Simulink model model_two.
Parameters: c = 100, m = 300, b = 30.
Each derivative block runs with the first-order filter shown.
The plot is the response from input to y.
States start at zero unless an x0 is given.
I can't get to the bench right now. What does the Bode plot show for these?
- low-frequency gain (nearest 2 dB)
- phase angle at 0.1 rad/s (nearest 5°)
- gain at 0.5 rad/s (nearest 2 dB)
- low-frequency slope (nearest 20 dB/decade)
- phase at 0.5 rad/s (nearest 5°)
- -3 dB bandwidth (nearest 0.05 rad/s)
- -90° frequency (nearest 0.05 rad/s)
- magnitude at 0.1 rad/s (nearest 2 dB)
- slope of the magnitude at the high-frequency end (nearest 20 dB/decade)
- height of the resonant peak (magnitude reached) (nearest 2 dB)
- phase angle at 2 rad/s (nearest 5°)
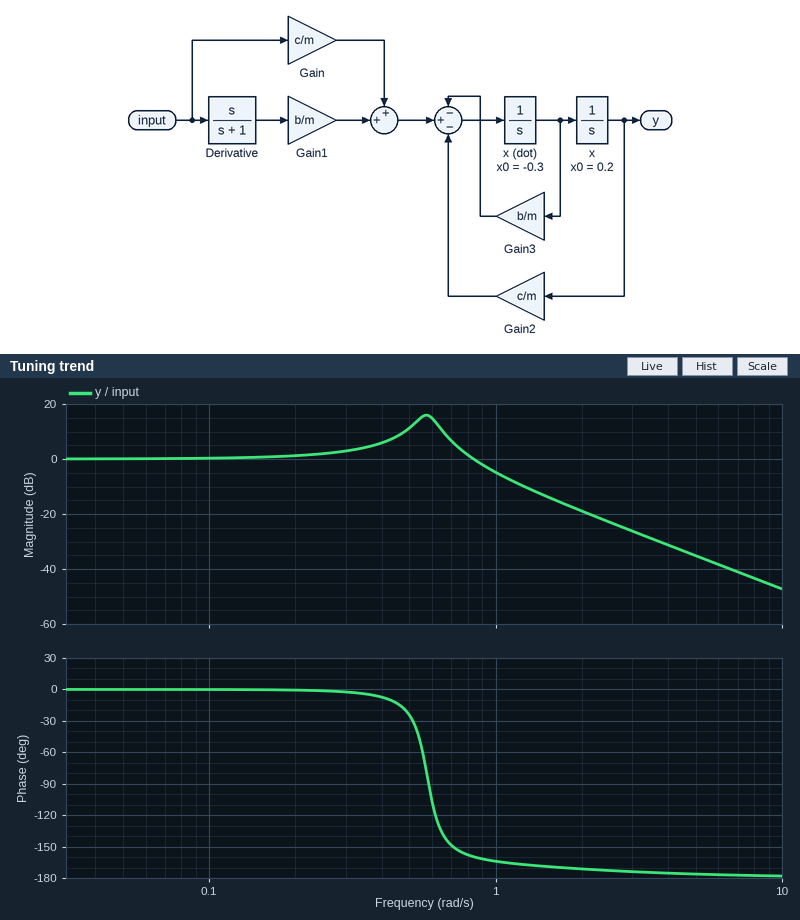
0 dB
0°
12 dB
0 dB/decade
-25°
0.95 rad/s
0.60 rad/s
0 dB
-40 dB/decade
16 dB
-170°
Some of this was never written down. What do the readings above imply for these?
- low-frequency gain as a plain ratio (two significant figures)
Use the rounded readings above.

1.0
